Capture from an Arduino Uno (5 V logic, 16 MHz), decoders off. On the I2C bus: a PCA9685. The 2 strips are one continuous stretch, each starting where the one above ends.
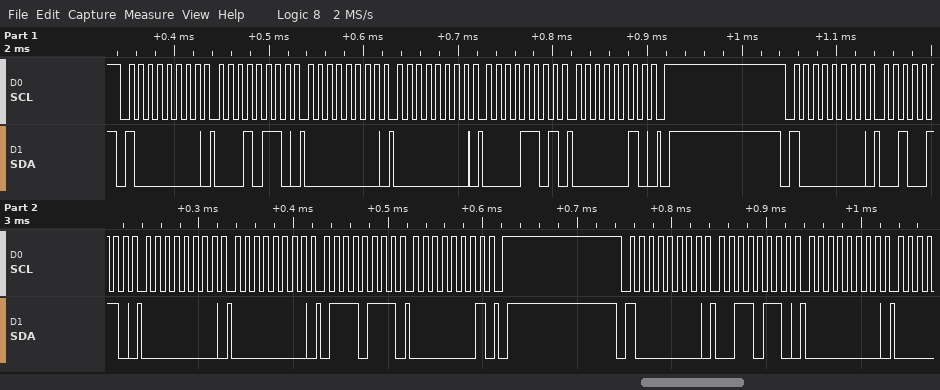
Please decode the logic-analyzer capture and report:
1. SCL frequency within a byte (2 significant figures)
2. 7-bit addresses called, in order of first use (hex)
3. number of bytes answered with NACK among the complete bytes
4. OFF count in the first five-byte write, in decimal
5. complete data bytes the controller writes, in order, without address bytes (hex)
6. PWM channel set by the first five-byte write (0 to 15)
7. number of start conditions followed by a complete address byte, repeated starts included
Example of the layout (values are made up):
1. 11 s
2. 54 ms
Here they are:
1. 100 kHz
2. 0x40
3. 0
4. 525
5. 16 00 00 0D 02 26 00 00 77 01 36 00
6. 4
7. 3
